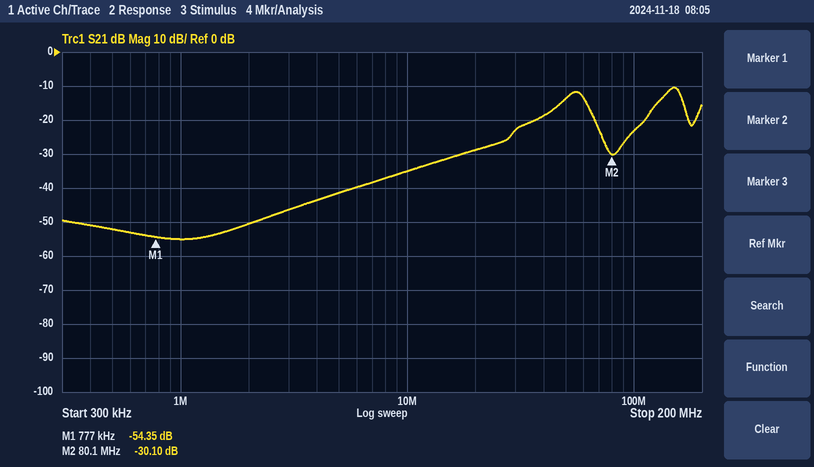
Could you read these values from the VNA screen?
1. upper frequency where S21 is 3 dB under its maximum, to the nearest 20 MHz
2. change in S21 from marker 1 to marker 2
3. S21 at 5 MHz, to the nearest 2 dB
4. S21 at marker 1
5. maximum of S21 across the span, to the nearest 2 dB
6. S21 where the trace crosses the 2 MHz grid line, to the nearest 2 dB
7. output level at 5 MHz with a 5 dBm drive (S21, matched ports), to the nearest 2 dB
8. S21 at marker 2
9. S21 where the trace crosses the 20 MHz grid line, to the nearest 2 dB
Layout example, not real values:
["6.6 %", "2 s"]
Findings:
["160 MHz", "24.25 dB", "-42 dB", "-54.35 dB", "-10 dB", "-50 dB", "-36 dBm", "-30.10 dB", "-28 dB"]
